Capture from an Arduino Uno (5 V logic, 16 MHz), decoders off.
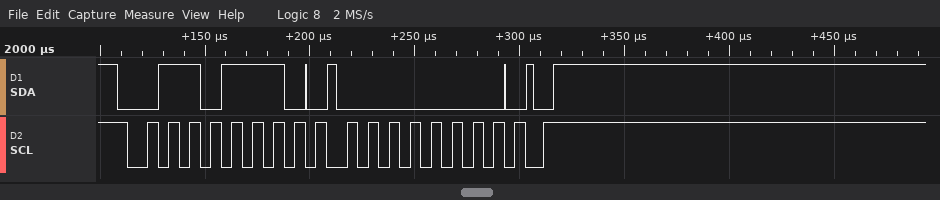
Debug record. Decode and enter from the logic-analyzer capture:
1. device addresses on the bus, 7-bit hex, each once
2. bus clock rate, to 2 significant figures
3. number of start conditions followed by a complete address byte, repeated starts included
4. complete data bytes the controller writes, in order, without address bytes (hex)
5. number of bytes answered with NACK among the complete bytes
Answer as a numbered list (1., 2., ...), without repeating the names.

1. 0x37
2. 100 kHz
3. 1
4. 00
5. 0
